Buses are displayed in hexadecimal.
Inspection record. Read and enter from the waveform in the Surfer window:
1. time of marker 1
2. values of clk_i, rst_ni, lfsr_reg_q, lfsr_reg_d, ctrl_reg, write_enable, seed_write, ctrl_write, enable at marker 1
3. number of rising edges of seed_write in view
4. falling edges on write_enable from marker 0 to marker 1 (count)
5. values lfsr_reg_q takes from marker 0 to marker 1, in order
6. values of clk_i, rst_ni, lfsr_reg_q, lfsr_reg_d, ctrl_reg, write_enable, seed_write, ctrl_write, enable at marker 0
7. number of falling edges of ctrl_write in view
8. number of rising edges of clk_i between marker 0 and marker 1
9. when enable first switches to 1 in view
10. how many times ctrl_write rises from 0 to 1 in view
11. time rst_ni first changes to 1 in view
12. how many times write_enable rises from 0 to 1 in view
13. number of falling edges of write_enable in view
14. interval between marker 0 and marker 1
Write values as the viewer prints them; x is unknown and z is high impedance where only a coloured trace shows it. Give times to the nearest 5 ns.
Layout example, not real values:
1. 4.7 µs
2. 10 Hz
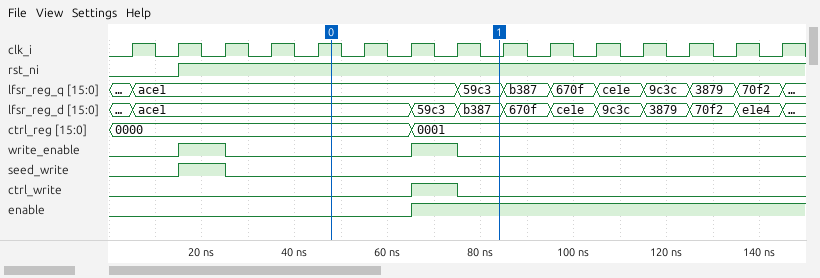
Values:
1. 85 ns
2. clk_i=0, rst_ni=1, lfsr_reg_q=59c3, lfsr_reg_d=b387, ctrl_reg=0001, write_enable=0, seed_write=0, ctrl_write=0, enable=1
3. 1
4. 1
5. ace1, 59c3
6. clk_i=1, rst_ni=1, lfsr_reg_q=ace1, lfsr_reg_d=ace1, ctrl_reg=0000, write_enable=0, seed_write=0, ctrl_write=0, enable=0
7. 1
8. 3
9. 65 ns
10. 1
11. 15 ns
12. 2
13. 2
14. 35 ns
